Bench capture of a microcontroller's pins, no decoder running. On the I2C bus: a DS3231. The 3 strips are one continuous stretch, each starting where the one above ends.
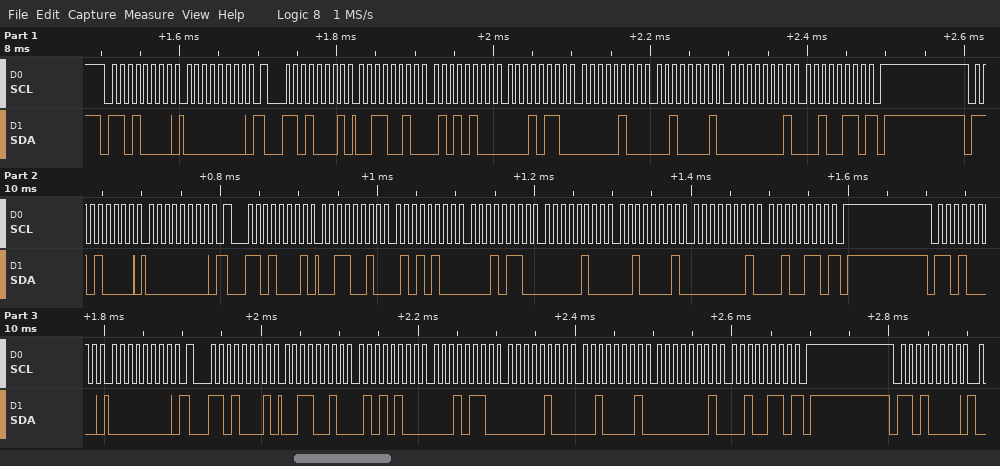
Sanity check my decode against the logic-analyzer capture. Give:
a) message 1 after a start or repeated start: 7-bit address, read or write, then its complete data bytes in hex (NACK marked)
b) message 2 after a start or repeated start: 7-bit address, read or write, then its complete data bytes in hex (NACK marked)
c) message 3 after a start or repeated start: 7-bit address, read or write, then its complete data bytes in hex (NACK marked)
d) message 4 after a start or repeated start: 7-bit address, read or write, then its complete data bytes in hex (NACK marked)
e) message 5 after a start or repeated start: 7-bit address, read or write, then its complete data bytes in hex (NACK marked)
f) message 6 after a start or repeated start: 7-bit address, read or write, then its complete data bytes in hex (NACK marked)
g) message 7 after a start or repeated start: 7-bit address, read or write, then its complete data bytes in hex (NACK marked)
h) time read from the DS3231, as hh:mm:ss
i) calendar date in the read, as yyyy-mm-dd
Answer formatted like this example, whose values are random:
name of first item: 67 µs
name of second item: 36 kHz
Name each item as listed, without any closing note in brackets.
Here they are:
message 1 after a start or repeated start: 7-bit address, read or write, then its complete data bytes in hex: 0x68 write: 00
message 2 after a start or repeated start: 7-bit address, read or write, then its complete data bytes in hex: 0x68 read: 32 54 16 04 21 01 26 NACK
message 3 after a start or repeated start: 7-bit address, read or write, then its complete data bytes in hex: 0x68 write: 00
message 4 after a start or repeated start: 7-bit address, read or write, then its complete data bytes in hex: 0x68 read: 32 54 16 04 21 01 26 NACK
message 5 after a start or repeated start: 7-bit address, read or write, then its complete data bytes in hex: 0x68 write: 00
message 6 after a start or repeated start: 7-bit address, read or write, then its complete data bytes in hex: 0x68 read: 32 54 16 04 21 01 26 NACK
message 7 after a start or repeated start: 7-bit address, read or write, then its complete data bytes in hex: 0x68 write
time read from the DS3231, as hh:mm:ss: 16:54:32
calendar date in the read, as yyyy-mm-dd: 2026-01-21
